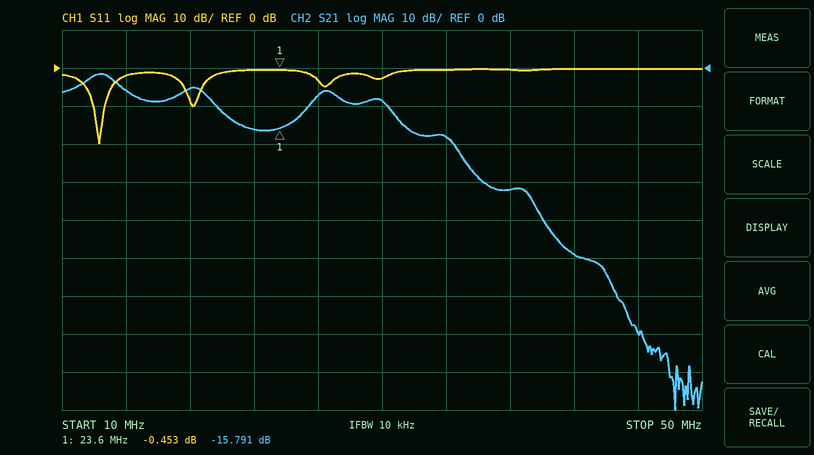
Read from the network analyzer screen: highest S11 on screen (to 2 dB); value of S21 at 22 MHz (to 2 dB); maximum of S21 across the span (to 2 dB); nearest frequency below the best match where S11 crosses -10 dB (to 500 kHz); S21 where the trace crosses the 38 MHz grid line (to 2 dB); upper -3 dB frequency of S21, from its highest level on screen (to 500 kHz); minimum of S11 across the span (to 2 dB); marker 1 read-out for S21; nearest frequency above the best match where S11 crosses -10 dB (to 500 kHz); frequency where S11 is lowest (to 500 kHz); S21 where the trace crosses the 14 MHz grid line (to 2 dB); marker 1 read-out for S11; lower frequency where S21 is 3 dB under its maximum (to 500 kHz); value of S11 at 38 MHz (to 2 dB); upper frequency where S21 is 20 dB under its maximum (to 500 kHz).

0 dB
-16 dB
-2 dB
12.0 MHz
-32 dB
13.5 MHz
-20 dB
-15.791 dB
12.5 MHz
12.5 MHz
-6 dB
-0.453 dB
11.0 MHz
0 dB
34.5 MHz
